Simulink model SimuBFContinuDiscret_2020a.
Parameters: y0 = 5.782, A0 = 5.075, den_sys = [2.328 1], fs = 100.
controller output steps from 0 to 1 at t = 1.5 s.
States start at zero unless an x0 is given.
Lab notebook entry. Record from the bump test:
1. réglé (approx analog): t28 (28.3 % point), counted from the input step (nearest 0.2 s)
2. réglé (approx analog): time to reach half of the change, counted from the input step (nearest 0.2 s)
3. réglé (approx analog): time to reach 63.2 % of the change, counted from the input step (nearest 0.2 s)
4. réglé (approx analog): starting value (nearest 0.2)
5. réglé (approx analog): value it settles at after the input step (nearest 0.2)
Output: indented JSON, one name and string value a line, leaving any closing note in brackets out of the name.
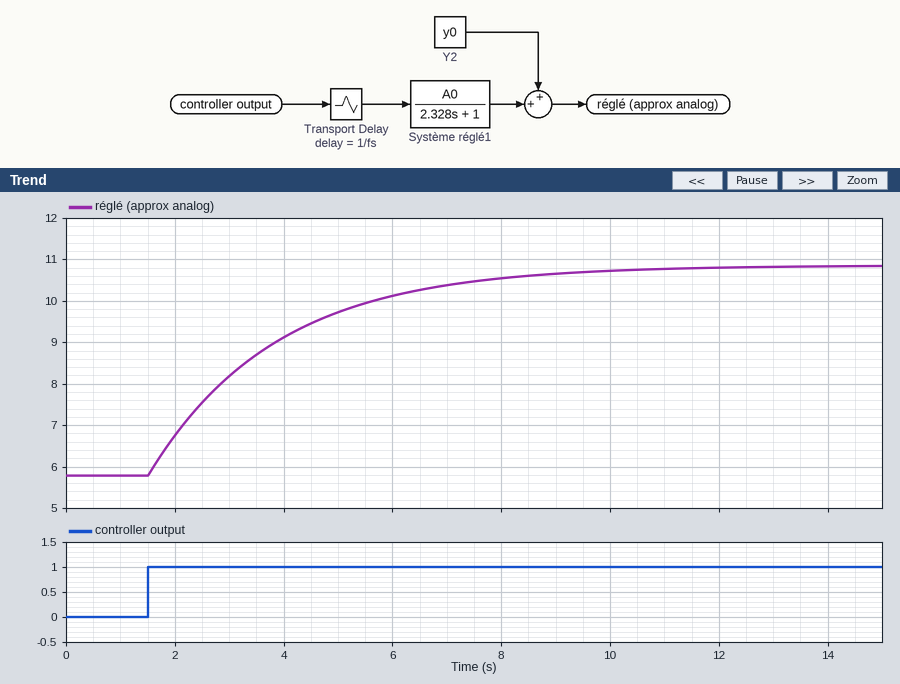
{
  "réglé (approx analog): t28 (28.3 % point), counted from the input step": "0.8 s",
  "réglé (approx analog): time to reach half of the change, counted from the input step": "1.6 s",
  "réglé (approx analog): time to reach 63.2 % of the change, counted from the input step": "2.4 s",
  "réglé (approx analog): starting value": "5.8",
  "réglé (approx analog): value it settles at after the input step": "10.8"
}
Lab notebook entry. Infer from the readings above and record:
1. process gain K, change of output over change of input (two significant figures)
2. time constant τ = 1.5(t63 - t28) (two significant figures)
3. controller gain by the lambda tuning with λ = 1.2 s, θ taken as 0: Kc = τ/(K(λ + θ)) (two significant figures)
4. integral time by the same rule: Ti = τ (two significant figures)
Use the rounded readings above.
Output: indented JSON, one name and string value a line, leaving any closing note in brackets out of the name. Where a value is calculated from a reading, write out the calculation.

{
  "process gain K, change of output over change of input": "(10.8 - 5.8) / 1 = 5.0",
  "time constant τ = 1.5(t63 - t28)": "1.5 × (2.4 - 0.8) = 2.4 s",
  "controller gain by the lambda tuning with λ = 1.2 s, θ taken as 0: Kc = τ/(K(λ + θ))": "2.4 / (5 × (1.2 + 0)) = 0.40",
  "integral time by the same rule: Ti = τ": "2.4 s"
}
